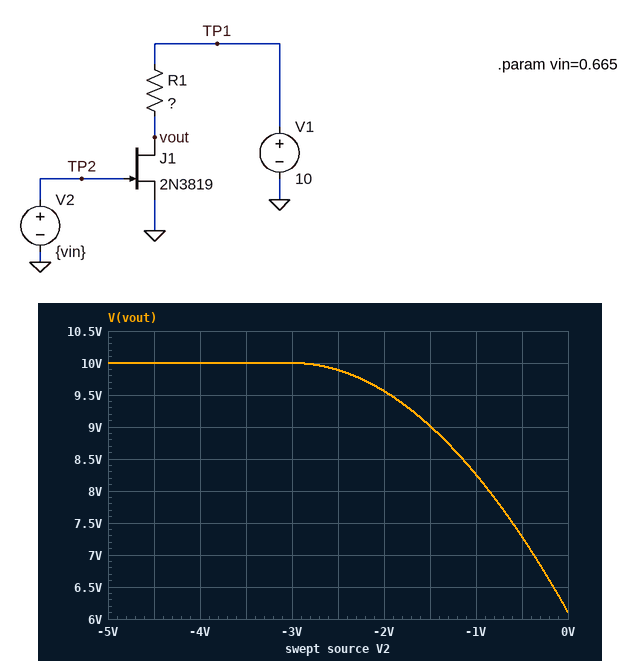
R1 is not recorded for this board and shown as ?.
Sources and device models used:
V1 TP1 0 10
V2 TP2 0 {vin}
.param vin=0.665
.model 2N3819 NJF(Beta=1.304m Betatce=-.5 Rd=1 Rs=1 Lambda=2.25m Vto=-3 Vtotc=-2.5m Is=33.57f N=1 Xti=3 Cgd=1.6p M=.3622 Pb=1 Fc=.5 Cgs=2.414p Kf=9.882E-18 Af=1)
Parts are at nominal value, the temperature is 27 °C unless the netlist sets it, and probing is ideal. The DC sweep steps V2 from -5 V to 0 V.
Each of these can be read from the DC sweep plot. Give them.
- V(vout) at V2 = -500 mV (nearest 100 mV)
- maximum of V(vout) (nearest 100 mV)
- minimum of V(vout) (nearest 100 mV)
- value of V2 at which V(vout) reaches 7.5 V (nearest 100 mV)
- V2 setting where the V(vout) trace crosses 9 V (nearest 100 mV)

7.3 V
10.0 V
6.1 V
-600 mV
-1.5 V
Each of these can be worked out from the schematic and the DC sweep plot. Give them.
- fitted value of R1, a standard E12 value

330 Ω
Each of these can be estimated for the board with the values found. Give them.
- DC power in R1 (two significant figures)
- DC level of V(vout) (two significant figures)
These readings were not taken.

100 mW
4.2 V
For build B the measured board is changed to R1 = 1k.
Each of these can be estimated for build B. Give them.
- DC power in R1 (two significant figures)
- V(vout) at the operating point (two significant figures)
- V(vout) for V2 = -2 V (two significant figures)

79 mW
1.1 V
8.7 V
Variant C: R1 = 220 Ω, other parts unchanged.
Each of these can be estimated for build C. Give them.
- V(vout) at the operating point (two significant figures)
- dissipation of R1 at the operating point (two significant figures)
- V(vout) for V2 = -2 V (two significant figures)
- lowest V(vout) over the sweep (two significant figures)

6.1 V
68 mW
9.7 V
7.4 V
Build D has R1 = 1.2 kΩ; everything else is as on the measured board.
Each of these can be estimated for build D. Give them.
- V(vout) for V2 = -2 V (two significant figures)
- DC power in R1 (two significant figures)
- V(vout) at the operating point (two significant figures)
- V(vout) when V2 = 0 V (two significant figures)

8.4 V
69 mW
920 mV
1.2 V
